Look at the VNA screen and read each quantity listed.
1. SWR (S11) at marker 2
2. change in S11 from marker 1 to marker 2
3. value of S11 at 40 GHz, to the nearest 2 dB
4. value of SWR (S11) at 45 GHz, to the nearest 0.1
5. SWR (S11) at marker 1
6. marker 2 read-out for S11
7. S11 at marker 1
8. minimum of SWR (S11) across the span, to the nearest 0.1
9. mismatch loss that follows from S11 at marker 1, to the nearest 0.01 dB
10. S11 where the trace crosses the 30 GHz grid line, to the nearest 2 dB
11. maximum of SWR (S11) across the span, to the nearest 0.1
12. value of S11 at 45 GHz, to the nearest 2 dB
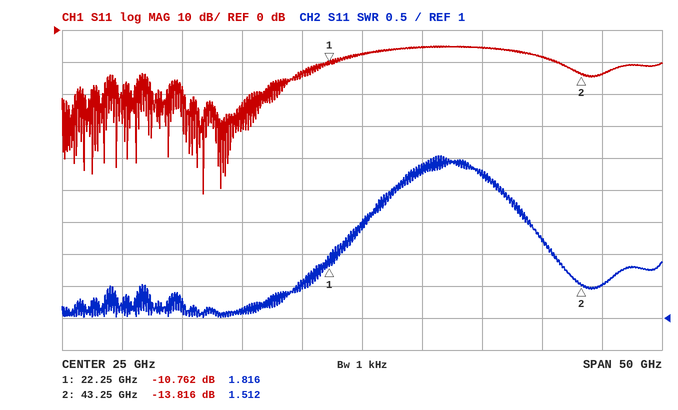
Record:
1.512
-3.054 dB
-8 dB
1.5
1.816
-13.816 dB
-10.762 dB
1.0
0.38 dB
-6 dB
3.5
-14 dB
